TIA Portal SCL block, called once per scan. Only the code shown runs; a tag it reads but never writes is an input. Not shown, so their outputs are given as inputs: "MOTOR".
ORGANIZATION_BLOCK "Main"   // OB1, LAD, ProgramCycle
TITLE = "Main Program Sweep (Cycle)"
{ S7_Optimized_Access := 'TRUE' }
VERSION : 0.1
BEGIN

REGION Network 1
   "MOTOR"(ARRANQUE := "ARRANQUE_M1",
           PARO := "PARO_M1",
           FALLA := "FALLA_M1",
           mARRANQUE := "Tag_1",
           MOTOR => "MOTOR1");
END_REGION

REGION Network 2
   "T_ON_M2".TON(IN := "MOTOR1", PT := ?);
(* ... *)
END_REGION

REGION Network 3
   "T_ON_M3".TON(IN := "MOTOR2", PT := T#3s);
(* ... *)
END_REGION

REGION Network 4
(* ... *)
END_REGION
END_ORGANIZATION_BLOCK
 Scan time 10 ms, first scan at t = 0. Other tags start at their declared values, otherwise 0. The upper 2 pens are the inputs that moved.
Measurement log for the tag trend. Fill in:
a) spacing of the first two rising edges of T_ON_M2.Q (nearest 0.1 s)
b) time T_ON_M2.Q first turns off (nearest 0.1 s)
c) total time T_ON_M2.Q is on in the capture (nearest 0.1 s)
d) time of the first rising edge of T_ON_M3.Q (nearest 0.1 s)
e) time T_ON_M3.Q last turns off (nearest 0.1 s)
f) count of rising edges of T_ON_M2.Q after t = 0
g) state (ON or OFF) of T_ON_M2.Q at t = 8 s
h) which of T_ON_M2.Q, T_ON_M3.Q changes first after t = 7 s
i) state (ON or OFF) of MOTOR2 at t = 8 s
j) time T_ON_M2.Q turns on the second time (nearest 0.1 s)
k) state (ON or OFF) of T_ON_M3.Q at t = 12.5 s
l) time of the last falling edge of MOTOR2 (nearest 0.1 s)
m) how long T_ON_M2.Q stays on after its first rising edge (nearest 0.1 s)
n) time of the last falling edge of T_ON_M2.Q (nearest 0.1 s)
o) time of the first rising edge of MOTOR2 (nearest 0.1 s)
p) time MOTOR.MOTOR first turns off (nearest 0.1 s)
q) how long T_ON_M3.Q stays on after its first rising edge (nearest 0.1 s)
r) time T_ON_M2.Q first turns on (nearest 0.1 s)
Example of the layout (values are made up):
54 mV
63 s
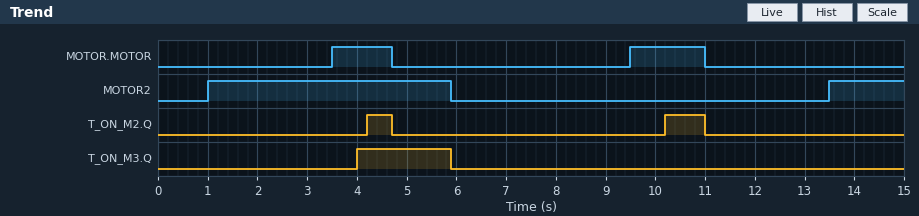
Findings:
6.0 s
4.7 s
1.3 s
4.0 s
5.9 s
2
OFF
T_ON_M2.Q
OFF
10.2 s
OFF
5.9 s
0.5 s
11.0 s
1.0 s
4.7 s
1.9 s
4.2 s
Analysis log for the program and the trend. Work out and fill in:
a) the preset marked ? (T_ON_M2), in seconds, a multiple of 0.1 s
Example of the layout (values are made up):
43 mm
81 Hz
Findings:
0.7 s
